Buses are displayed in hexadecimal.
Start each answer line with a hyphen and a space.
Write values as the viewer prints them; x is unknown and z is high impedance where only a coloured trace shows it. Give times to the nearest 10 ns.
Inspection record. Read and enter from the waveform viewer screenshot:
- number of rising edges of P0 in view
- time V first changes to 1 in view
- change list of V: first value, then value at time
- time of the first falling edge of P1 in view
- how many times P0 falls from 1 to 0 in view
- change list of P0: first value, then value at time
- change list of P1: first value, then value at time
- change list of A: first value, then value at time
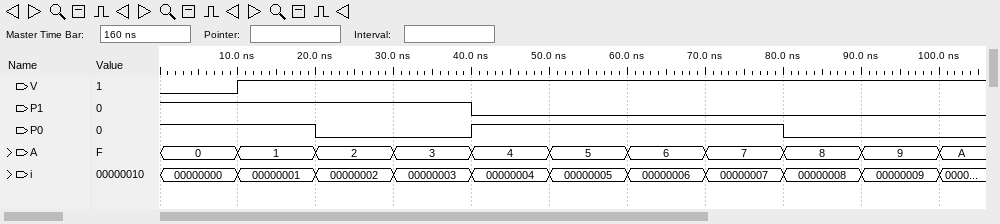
- 1
- 10 ns
- 0, 1 at 10 ns
- 40 ns
- 2
- 1, 0 at 20 ns, 1 at 40 ns, 0 at 80 ns
- 1, 0 at 40 ns
- 0, 1 at 10 ns, 2 at 20 ns, 3 at 30 ns, 4 at 40 ns, 5 at 50 ns, 6 at 60 ns, 7 at 70 ns, 8 at 80 ns, 9 at 90 ns, A at 100 ns
